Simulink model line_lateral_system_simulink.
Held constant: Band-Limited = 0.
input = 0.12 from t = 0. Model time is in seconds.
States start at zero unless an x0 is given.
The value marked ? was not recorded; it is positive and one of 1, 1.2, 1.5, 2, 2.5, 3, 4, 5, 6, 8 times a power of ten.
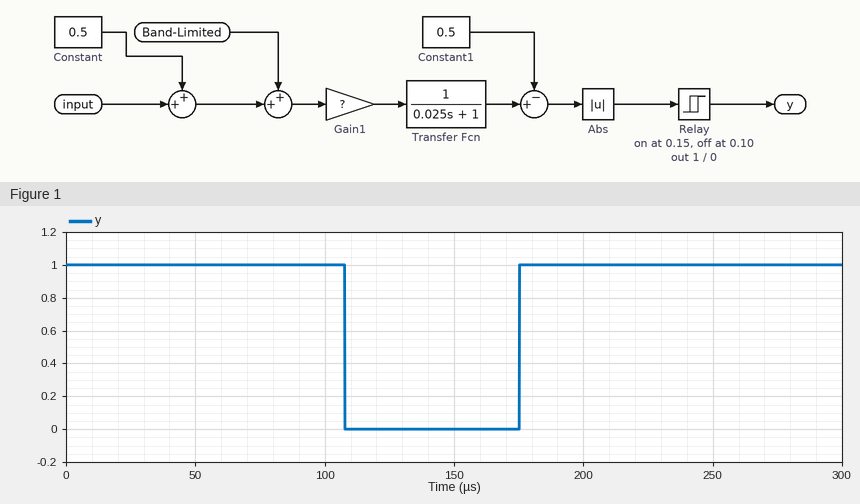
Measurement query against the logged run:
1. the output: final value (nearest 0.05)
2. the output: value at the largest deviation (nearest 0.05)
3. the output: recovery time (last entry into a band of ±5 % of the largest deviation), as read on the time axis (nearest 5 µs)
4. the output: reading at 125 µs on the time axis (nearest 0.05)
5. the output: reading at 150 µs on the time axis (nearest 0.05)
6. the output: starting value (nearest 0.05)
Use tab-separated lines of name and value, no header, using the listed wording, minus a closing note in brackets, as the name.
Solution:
the output: final value	1.00
the output: value at the largest deviation	0.00
the output: recovery time (last entry into a band of ±5 % of the largest deviation), as read on the time axis	175 µs
the output: reading at 125 µs on the time axis	0.00
the output: reading at 150 µs on the time axis	0.00
the output: starting value	1.00
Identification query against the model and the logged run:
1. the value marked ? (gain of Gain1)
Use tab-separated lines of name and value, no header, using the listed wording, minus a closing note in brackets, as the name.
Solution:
the value marked ?	150
